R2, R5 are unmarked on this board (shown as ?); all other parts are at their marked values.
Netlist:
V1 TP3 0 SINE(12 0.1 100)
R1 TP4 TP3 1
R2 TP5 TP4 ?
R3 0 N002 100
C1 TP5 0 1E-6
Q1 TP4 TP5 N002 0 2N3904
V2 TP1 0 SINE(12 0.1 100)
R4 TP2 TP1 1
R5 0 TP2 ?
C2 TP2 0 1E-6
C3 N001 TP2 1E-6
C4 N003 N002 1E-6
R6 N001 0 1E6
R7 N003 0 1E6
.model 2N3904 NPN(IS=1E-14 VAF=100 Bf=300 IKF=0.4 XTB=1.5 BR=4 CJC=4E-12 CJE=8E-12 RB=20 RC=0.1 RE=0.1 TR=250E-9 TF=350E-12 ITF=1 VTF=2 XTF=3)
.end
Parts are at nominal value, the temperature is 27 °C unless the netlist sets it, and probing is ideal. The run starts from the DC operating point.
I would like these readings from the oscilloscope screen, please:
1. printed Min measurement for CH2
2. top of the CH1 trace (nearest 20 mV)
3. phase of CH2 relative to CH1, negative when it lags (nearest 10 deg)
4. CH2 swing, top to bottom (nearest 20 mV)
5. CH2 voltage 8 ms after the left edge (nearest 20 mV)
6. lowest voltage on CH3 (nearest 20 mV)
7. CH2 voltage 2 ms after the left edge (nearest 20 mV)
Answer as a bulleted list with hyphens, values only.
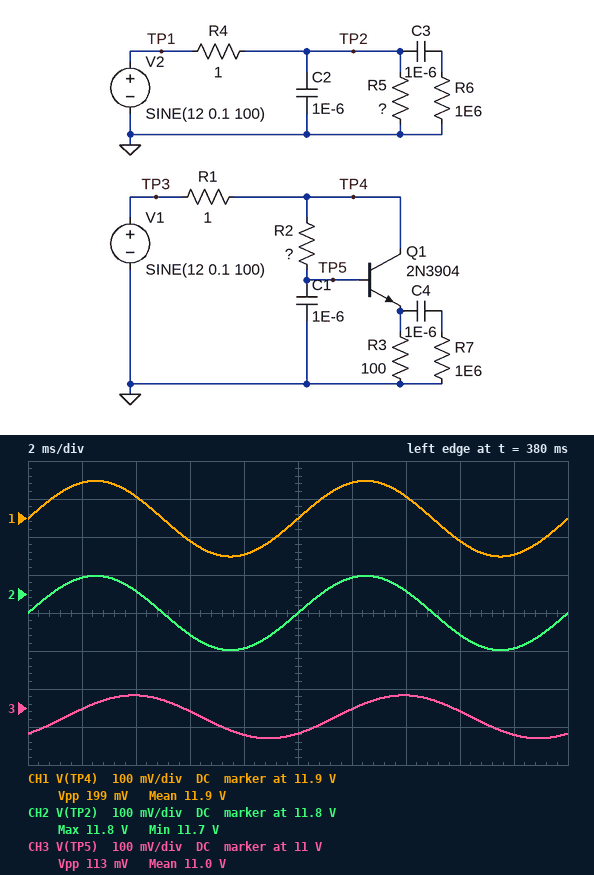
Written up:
- 11.7 V
- 12.00 V
- 0 deg
- 200 mV
- 11.66 V
- 10.92 V
- 11.84 V
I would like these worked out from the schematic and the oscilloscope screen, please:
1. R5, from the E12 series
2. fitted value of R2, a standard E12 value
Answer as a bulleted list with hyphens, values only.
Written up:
- 47 Ω
- 2.2 kΩ
